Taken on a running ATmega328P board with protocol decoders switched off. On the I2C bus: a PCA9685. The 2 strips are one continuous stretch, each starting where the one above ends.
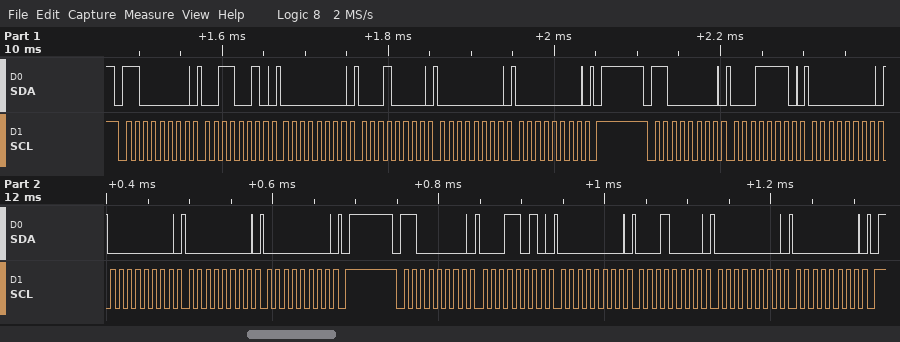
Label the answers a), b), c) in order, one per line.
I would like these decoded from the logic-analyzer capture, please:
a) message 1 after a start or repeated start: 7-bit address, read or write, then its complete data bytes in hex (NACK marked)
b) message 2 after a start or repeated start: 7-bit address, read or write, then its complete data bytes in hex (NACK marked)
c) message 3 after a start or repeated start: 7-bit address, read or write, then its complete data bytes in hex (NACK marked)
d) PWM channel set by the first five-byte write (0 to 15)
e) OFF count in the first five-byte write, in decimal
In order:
a) 0x60 write: 32 00 10 00 00
b) 0x60 write: 1E 00 00 00 00
c) 0x60 write: 1A 00 10 00 00
d) 11
e) 0
